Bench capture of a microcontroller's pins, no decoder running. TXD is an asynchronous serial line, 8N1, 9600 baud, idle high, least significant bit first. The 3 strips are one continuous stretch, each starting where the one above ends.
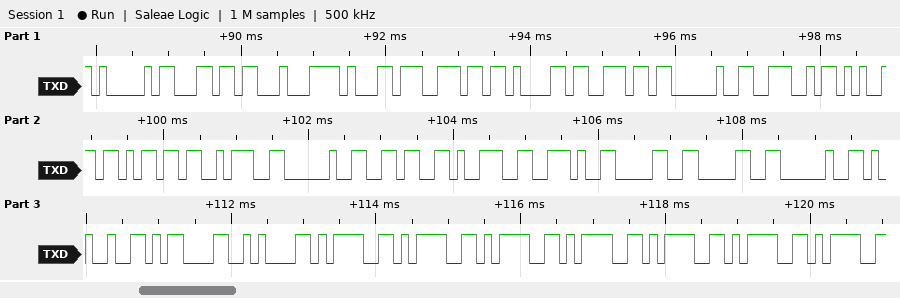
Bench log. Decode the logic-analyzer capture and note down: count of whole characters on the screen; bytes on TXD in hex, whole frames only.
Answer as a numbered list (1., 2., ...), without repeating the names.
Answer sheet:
1. 29
2. 41 6C C4 B1 6E 61 6E 20 4E 65 6D 3A 20 36 39 2E 30 30 20 25 0D 0A 3D 3D 3D 3D 3D 3D 3D
